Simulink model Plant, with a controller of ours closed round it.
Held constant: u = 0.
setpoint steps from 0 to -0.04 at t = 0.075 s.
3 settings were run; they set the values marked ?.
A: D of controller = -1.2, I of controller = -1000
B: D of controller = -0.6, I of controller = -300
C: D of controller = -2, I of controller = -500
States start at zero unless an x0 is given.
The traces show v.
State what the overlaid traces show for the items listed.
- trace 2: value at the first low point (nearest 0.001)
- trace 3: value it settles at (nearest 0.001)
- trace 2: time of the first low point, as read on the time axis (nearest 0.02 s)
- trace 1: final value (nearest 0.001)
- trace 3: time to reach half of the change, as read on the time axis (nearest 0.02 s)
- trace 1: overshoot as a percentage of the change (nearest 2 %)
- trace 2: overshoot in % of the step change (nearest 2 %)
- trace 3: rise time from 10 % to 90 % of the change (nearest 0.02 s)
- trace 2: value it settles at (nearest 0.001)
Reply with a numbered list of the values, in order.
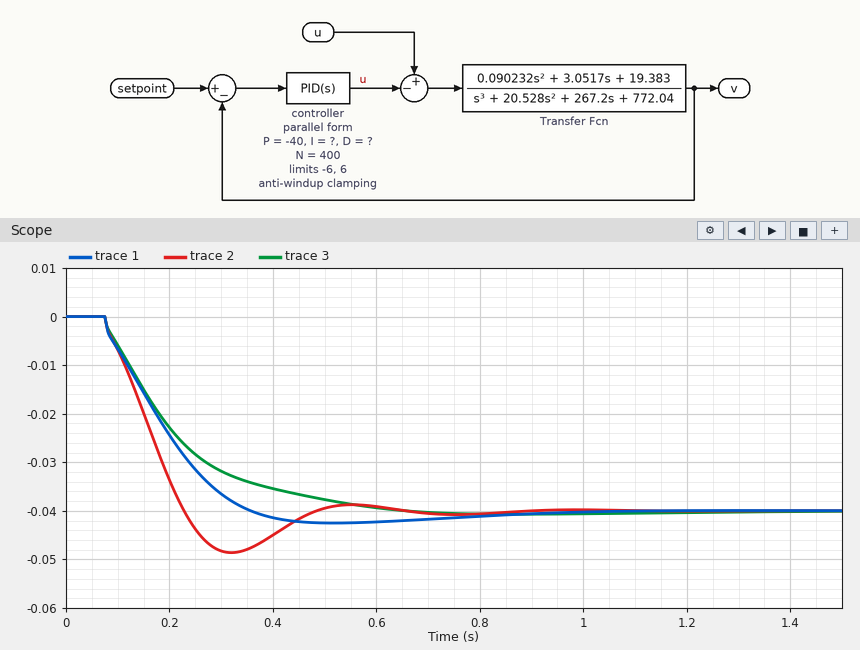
1. -0.049
2. -0.040
3. 0.32 s
4. -0.040
5. 0.18 s
6. 6 %
7. 22 %
8. 0.34 s
9. -0.040
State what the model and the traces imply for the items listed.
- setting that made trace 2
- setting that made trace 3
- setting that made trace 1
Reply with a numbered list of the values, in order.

1. A
2. B
3. C
